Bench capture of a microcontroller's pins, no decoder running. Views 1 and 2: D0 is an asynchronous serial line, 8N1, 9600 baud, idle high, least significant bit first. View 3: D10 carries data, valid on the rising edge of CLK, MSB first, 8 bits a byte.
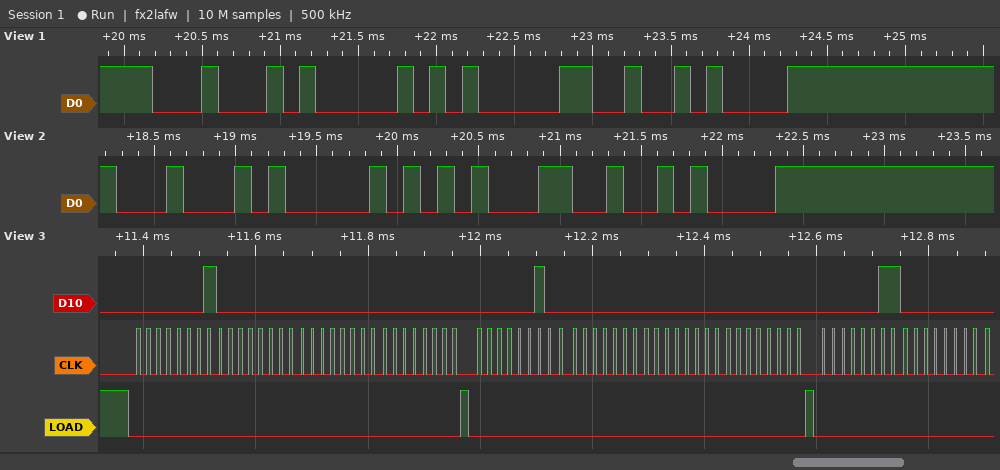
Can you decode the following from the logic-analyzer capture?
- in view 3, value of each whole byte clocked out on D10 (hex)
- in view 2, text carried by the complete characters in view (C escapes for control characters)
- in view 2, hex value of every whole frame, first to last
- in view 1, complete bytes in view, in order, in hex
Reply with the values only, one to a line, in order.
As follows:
0x01 0x00 0x00 0x00 0x02 0x00 0x00 0x00 0x03 0x00
"DP1\n"
44 50 31 0A
44 50 30 0A
